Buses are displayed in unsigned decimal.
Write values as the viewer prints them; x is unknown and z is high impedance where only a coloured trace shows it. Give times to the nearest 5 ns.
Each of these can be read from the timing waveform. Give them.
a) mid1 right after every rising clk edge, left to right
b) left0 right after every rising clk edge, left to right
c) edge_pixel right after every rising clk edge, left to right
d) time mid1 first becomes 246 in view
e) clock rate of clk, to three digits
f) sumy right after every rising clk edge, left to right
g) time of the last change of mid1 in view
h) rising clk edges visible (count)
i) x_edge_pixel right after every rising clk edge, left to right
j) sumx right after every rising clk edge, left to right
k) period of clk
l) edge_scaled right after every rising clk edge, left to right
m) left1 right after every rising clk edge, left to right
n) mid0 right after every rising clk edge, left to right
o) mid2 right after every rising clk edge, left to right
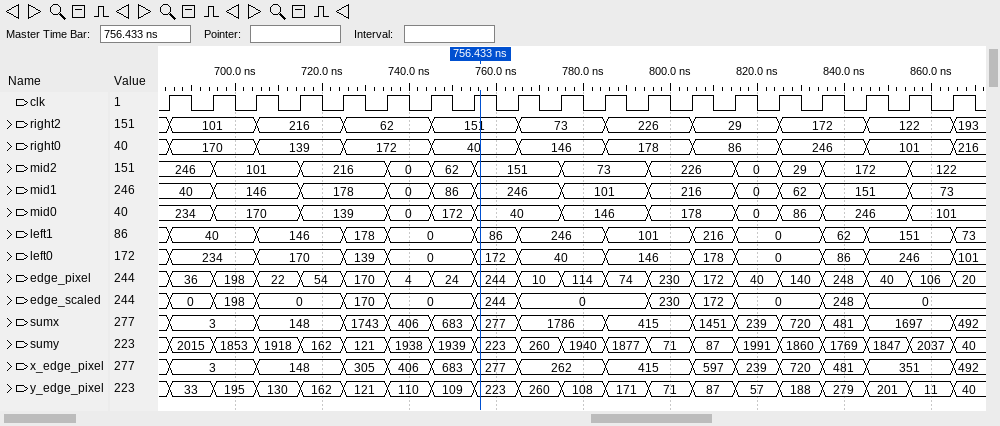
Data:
40, 146, 146, 178, 178, 0, 86, 246, 246, 101, 101, 216, 216, 0, 62, 151, 151, 73, 73
234, 234, 170, 170, 139, 0, 0, 172, 40, 40, 146, 146, 178, 0, 0, 86, 246, 246, 101
36, 198, 22, 54, 170, 4, 24, 244, 10, 114, 74, 230, 172, 40, 140, 248, 40, 106, 20
755 ns
100 MHz
2015, 1853, 1918, 162, 121, 1938, 1939, 223, 260, 1940, 1877, 71, 87, 1991, 1860, 1769, 1847, 2037, 40
855 ns
19
3, 3, 148, 148, 305, 406, 683, 277, 262, 262, 415, 415, 597, 239, 720, 481, 351, 351, 492
3, 3, 148, 148, 1743, 406, 683, 277, 1786, 1786, 415, 415, 1451, 239, 720, 481, 1697, 1697, 492
10 ns
0, 198, 0, 0, 170, 0, 0, 244, 0, 0, 0, 230, 172, 0, 0, 248, 0, 0, 0
40, 40, 146, 146, 178, 0, 0, 86, 246, 246, 101, 101, 216, 0, 0, 62, 151, 151, 73
234, 170, 170, 139, 139, 0, 172, 40, 40, 146, 146, 178, 178, 0, 86, 246, 246, 101, 101
246, 101, 101, 216, 216, 0, 62, 151, 151, 73, 73, 226, 226, 0, 29, 172, 172, 122, 122
